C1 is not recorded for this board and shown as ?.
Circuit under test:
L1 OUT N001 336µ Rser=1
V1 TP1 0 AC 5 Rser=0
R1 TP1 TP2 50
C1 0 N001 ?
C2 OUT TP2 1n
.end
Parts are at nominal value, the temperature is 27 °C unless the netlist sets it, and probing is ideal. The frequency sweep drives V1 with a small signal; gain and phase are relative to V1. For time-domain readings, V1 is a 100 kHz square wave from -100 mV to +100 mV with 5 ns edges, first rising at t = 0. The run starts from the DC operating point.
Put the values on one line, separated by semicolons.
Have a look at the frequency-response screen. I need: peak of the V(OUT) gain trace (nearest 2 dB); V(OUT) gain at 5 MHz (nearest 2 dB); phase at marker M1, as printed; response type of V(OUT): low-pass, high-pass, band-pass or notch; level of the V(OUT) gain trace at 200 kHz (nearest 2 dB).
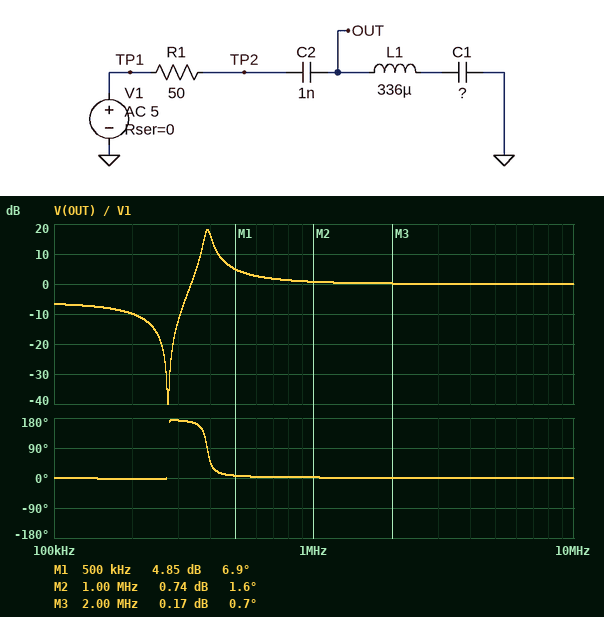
18 dB; 0 dB; 6.9 deg; band-pass; -10 dB
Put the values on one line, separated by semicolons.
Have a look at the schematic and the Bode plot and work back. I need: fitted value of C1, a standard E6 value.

1 nF
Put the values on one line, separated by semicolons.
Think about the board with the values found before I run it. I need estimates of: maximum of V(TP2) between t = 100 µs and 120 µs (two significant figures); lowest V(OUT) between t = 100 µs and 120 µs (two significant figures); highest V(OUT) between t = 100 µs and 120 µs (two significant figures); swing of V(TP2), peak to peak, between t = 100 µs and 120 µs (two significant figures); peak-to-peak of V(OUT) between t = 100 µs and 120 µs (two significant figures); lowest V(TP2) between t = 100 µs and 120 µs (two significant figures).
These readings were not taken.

110 mV; -59 mV; 160 mV; 210 mV; 220 mV; -110 mV
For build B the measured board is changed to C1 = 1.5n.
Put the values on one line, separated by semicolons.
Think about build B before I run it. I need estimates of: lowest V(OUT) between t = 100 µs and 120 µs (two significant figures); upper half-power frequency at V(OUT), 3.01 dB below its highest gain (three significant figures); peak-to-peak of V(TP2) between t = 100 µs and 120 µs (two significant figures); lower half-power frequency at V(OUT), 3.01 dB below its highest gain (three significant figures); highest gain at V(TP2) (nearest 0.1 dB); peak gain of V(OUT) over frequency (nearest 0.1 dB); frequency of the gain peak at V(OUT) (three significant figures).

-77 mV; 369 kHz; 220 mV; 344 kHz; 0 dB; 18.9 dB; 355 kHz
